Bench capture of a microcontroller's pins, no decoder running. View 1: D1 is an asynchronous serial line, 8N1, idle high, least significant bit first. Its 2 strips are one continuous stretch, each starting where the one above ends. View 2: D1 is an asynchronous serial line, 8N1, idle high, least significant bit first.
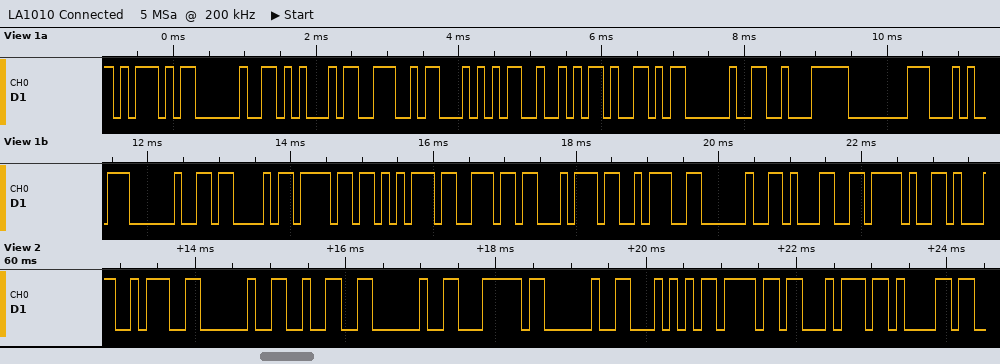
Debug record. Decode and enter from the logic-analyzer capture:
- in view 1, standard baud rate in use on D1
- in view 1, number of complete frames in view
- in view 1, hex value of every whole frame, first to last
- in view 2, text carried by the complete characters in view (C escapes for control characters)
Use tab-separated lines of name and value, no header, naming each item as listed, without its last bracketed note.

in view 1, standard baud rate in use on D1	9600 baud
in view 1, number of complete frames in view	21
in view 1, hex value of every whole frame, first to last	0x5D 0x20 0x45 0x4E 0x54 0x52 0x59 0x20 0xE2 0x80 0x94 0x20 0x43 0x6F 0x75 0x6E 0x74 0x3A 0x20 0x31 0x2F
in view 2, text carried by the complete characters in view	": 2 | Tota"
